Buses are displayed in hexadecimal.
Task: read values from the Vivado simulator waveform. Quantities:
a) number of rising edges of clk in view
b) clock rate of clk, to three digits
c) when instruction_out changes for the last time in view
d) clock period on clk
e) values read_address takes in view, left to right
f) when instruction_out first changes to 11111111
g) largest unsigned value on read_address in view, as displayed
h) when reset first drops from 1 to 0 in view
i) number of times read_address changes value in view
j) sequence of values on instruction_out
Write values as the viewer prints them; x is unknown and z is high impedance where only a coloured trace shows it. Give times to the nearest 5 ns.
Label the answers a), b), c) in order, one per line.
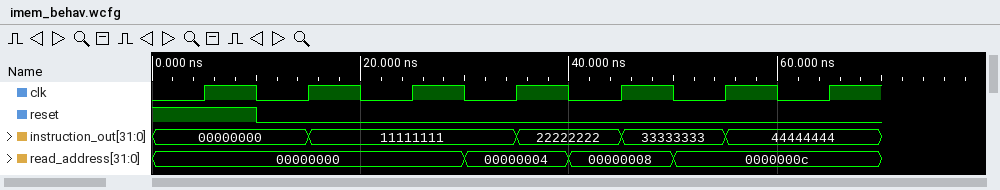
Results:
a) 7
b) 100 MHz
c) 55 ns
d) 10 ns
e) 00000000, 00000004, 00000008, 0000000c
f) 15 ns
g) 0000000c
h) 10 ns
i) 3
j) 00000000, 11111111, 22222222, 33333333, 44444444
